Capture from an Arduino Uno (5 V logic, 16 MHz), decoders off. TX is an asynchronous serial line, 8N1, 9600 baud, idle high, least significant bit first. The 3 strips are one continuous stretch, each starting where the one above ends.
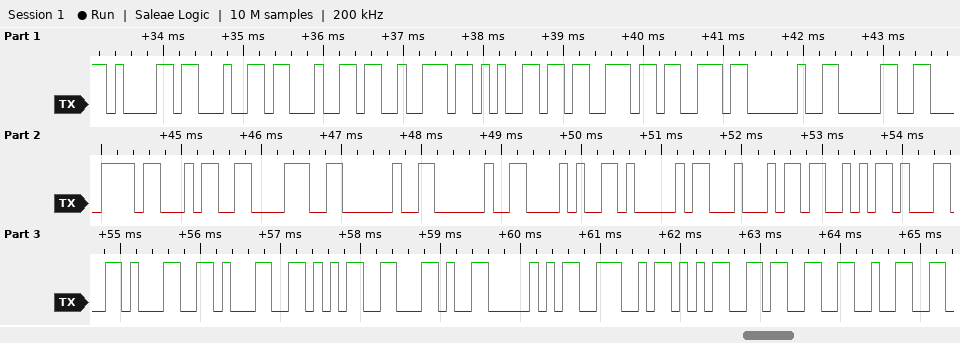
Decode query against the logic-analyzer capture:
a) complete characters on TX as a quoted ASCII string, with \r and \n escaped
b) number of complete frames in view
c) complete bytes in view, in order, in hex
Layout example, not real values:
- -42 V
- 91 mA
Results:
- "address 0x48  (ADS1115,PN532"
- 28
- 61 64 64 72 65 73 73 20 30 78 34 38 20 20 28 41 44 53 31 31 31 35 2C 50 4E 35 33 32
